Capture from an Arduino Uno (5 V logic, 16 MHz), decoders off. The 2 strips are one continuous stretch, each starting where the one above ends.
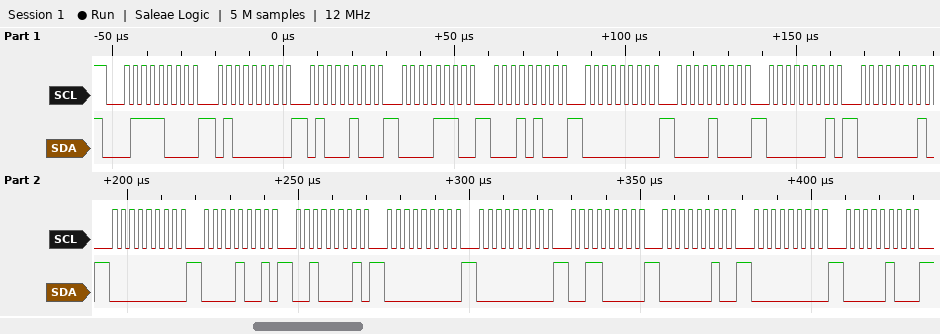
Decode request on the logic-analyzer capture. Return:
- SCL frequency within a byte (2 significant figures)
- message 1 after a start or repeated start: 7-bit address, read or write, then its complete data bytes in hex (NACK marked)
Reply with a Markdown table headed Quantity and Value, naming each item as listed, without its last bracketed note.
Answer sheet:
| Quantity | Value |
|---|---|
| SCL frequency within a byte | 400 kHz |
| message 1 after a start or repeated start: 7-bit address, read or write, then its complete data bytes in hex | 0x3C write: 40 44 0E 14 00 08 01 01 00 09 21 00 00 30 02 00 04 |
